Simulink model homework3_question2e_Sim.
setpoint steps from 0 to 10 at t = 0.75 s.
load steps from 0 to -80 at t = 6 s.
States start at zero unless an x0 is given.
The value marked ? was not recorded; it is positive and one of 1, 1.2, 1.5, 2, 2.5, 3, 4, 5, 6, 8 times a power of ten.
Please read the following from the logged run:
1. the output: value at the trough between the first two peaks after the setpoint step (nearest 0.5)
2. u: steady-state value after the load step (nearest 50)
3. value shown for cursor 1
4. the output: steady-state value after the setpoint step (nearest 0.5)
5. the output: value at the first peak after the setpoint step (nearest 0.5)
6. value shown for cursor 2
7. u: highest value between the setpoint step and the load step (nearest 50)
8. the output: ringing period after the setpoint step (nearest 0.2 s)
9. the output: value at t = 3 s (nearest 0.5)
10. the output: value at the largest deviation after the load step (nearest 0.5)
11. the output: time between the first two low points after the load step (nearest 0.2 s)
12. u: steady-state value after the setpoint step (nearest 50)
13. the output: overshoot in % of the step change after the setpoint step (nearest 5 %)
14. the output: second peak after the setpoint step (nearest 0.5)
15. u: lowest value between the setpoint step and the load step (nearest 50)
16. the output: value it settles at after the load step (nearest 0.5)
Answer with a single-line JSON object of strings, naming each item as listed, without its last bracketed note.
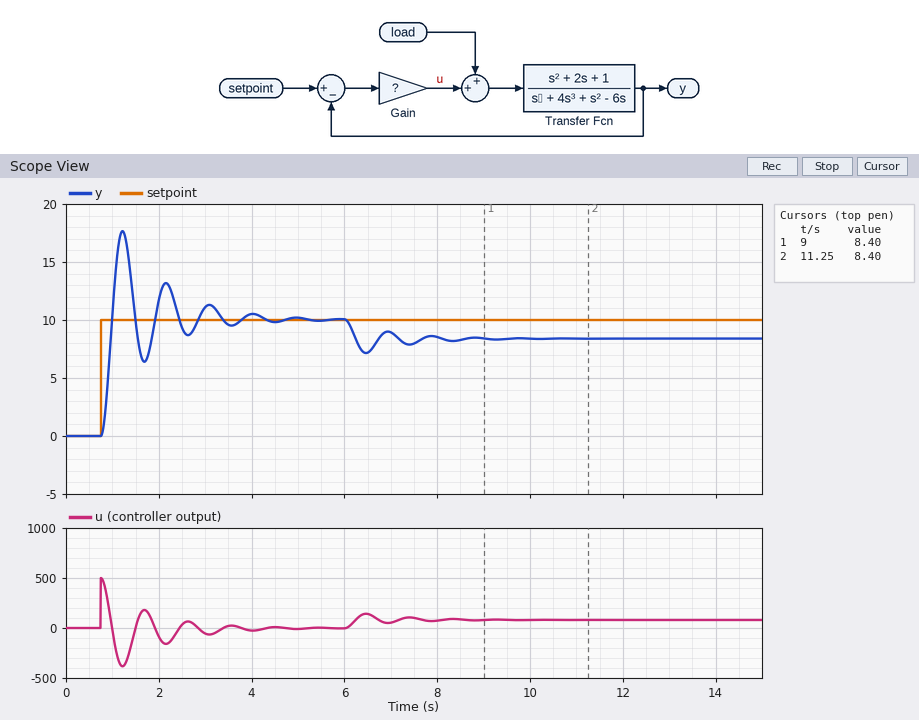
{"the output: value at the trough between the first two peaks after the setpoint step": "6.5", "u: steady-state value after the load step": "100", "value shown for cursor 1": "8.40", "the output: steady-state value after the setpoint step": "10.0", "the output: value at the first peak after the setpoint step": "17.5", "value shown for cursor 2": "8.40", "u: highest value between the setpoint step and the load step": "500", "the output: ringing period after the setpoint step": "1.0 s", "the output: value at t = 3 s": "11.0", "the output: value at the largest deviation after the load step": "7.0", "the output: time between the first two low points after the load step": "1.0 s", "u: steady-state value after the setpoint step": "0", "the output: overshoot in % of the step change after the setpoint step": "75 %", "the output: second peak after the setpoint step": "13.0", "u: lowest value between the setpoint step and the load step": "-400", "the output: value it settles at after the load step": "8.5"}
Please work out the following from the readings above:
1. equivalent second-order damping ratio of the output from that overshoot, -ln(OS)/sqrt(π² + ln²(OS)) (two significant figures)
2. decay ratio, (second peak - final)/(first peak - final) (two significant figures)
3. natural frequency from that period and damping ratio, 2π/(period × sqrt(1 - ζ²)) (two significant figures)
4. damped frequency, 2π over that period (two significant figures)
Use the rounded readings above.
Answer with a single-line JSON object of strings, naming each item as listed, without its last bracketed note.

{"equivalent second-order damping ratio of the output from that overshoot, -ln(OS)/sqrt(π² + ln²(OS))": "0.091", "decay ratio, (second peak - final)/(first peak - final)": "0.40", "natural frequency from that period and damping ratio, 2π/(period × sqrt(1 - ζ²))": "6.3 rad/s", "damped frequency, 2π over that period": "6.3 rad/s"}
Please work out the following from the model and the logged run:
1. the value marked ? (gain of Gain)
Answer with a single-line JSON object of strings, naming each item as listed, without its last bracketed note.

{"the value marked ?": "50"}
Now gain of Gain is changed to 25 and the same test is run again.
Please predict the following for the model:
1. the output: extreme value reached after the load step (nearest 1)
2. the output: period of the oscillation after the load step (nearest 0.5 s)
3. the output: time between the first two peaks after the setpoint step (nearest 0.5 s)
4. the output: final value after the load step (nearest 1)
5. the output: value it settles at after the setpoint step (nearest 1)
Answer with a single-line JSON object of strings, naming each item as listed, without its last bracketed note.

{"the output: extreme value reached after the load step": "4", "the output: period of the oscillation after the load step": "1.5 s", "the output: time between the first two peaks after the setpoint step": "1.5 s", "the output: final value after the load step": "7", "the output: value it settles at after the setpoint step": "10"}
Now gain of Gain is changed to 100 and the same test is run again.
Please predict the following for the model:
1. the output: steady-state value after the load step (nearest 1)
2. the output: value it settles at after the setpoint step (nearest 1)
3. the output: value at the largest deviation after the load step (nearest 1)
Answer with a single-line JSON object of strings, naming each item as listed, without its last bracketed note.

{"the output: steady-state value after the load step": "9", "the output: value it settles at after the setpoint step": "10", "the output: value at the largest deviation after the load step": "9"}
